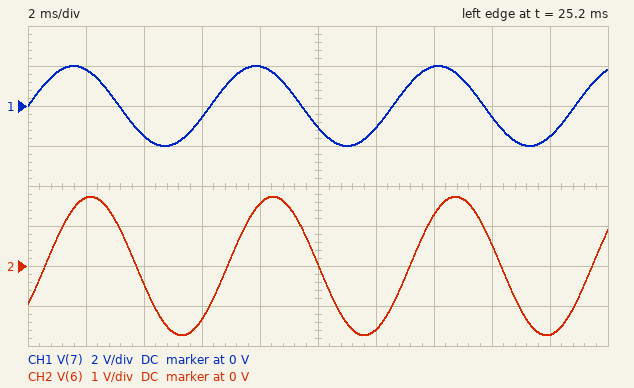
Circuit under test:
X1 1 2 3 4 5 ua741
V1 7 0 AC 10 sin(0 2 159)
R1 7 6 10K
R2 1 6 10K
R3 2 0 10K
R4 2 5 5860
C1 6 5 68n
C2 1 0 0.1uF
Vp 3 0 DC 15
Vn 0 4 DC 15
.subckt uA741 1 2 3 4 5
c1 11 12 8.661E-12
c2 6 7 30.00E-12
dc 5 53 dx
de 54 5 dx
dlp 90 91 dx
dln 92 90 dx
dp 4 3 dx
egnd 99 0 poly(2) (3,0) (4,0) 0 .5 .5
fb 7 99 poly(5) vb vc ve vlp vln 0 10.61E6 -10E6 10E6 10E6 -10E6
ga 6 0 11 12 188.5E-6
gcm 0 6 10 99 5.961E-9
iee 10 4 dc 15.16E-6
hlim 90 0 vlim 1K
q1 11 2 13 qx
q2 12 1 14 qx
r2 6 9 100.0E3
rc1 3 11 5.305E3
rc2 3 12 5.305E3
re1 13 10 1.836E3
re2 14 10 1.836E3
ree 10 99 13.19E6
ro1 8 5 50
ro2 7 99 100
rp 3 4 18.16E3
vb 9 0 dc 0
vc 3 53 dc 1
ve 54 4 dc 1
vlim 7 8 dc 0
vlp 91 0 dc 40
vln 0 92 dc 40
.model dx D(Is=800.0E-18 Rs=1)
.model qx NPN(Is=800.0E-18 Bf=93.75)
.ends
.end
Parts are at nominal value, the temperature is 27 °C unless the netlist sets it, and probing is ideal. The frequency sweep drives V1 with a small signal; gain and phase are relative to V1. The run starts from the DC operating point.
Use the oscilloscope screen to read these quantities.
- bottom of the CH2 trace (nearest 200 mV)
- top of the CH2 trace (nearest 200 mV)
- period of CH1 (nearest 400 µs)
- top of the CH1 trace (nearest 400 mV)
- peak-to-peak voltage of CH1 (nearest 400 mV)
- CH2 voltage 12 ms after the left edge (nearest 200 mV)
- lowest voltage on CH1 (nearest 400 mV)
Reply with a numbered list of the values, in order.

1. -1.8 V
2. 1.8 V
3. 6.4 ms
4. 2.0 V
5. 4.0 V
6. -1.6 V
7. -2.0 V
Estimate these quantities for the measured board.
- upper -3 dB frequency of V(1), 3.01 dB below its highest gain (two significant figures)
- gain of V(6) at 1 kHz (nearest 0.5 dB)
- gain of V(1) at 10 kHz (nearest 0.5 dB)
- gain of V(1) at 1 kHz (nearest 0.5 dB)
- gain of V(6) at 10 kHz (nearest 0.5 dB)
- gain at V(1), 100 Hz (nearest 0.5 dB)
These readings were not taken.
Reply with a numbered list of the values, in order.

1. 130 Hz
2. -13.0 dB
3. -68.5 dB
4. -29.0 dB
5. -32.5 dB
6. -2.0 dB
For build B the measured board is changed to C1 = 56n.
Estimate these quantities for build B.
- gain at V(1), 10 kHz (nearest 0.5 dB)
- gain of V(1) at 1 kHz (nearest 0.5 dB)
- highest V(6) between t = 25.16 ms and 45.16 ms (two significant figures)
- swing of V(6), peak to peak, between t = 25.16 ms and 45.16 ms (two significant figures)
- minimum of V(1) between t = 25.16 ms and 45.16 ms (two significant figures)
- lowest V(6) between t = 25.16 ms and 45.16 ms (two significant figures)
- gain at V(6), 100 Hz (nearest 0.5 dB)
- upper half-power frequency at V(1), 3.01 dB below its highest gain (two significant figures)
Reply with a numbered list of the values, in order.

1. -67.0 dB
2. -27.5 dB
3. 1.6 V
4. 3.3 V
5. -1.2 V
6. -1.6 V
7. -1.0 dB
8. 120 Hz
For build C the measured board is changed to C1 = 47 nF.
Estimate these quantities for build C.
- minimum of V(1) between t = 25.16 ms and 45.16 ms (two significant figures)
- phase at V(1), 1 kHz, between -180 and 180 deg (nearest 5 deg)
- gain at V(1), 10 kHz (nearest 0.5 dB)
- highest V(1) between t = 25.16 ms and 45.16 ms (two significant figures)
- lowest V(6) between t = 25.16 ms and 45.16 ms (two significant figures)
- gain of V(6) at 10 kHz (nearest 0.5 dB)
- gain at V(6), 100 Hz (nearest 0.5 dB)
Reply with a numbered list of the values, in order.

1. -1.1 V
2. -150 deg
3. -65.5 dB
4. 1.1 V
5. -1.6 V
6. -29.5 dB
7. -1.0 dB
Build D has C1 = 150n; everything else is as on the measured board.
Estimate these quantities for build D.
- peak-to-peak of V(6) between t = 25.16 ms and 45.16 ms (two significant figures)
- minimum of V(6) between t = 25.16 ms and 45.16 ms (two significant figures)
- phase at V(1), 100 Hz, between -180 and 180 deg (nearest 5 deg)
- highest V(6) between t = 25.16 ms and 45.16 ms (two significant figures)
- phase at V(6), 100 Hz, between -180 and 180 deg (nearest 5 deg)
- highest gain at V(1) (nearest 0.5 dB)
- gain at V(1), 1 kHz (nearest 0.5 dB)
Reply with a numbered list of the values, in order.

1. 4.6 V
2. -2.3 V
3. -60 deg
4. 2.3 V
5. -30 deg
6. 2.0 dB
7. -35.5 dB
